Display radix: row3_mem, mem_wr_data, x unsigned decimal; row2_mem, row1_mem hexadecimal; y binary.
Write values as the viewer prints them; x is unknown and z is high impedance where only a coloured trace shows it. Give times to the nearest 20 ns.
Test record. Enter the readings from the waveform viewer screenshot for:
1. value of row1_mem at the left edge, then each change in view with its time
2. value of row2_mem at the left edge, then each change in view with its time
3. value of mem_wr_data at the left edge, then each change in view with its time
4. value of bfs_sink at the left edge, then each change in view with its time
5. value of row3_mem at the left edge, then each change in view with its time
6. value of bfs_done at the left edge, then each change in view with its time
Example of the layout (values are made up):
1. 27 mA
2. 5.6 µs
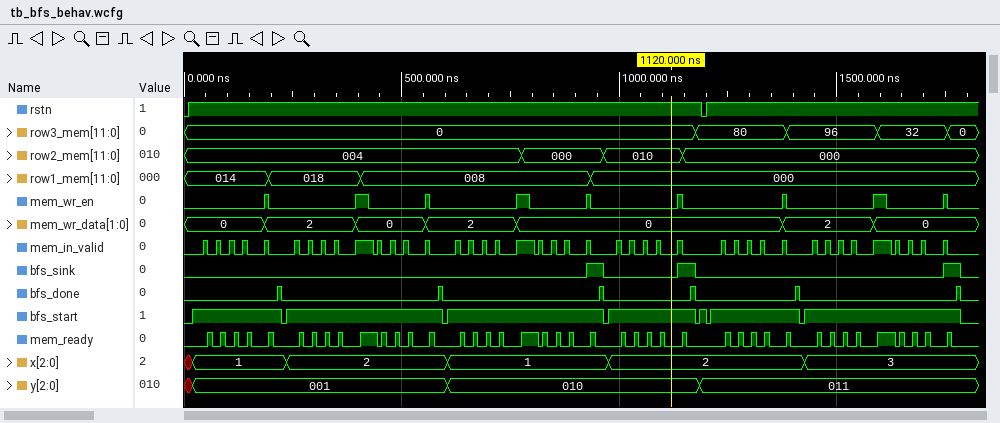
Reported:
1. 014, 018 at 200 ns, 008 at 400 ns, 000 at 940 ns
2. 004, 000 at 780 ns, 010 at 960 ns, 000 at 1140 ns
3. 0, 2 at 180 ns, 0 at 400 ns, 2 at 560 ns, 0 at 760 ns, 2 at 1380 ns, 0 at 1580 ns
4. 0, 1 at 920 ns, 0 at 960 ns, 1 at 1140 ns, 0 at 1180 ns, 1 at 1740 ns, 0 at 1780 ns
5. 0, 80 at 1180 ns, 96 at 1380 ns, 32 at 1600 ns, 0 at 1760 ns
6. 0, 1 at 220 ns, 0 at 220 ns, 1 at 580 ns, 0 at 600 ns, 1 at 960 ns, 0 at 960 ns, 1 at 1160 ns, 0 at 1180 ns, 1 at 1400 ns, 0 at 1420 ns, 1 at 1780 ns, 0 at 1780 ns
